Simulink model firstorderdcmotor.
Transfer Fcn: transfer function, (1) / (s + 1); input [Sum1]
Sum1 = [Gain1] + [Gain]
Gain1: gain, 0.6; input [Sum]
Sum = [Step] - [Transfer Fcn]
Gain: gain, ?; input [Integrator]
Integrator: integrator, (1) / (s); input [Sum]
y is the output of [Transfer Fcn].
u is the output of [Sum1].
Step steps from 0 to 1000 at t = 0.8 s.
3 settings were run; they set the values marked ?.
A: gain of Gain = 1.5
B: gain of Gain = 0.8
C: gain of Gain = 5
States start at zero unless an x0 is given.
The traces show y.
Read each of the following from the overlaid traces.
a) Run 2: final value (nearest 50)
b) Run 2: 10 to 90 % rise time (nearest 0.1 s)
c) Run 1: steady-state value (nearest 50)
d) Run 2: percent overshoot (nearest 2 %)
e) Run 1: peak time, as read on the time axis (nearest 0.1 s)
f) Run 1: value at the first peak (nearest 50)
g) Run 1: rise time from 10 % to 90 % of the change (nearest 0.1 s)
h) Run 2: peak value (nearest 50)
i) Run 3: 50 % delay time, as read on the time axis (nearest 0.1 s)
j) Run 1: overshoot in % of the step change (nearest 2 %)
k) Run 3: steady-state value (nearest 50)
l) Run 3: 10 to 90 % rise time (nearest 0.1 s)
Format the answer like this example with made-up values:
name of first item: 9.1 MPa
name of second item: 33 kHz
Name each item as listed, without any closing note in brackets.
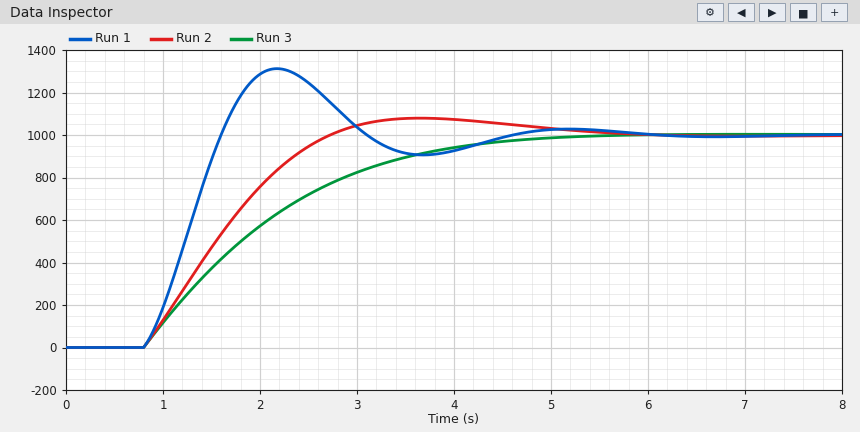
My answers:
Run 2: final value: 1000
Run 2: 10 to 90 % rise time: 1.4 s
Run 1: steady-state value: 1000
Run 2: percent overshoot: 8 %
Run 1: peak time, as read on the time axis: 2.2 s
Run 1: value at the first peak: 1300
Run 1: rise time from 10 % to 90 % of the change: 0.6 s
Run 2: peak value: 1100
Run 3: 50 % delay time, as read on the time axis: 1.8 s
Run 1: overshoot in % of the step change: 32 %
Run 3: steady-state value: 1000
Run 3: 10 to 90 % rise time: 2.6 s
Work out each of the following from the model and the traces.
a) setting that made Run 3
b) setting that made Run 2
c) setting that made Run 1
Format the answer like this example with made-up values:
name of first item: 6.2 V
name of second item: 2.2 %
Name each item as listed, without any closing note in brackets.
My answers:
setting that made Run 3: B
setting that made Run 2: A
setting that made Run 1: C
